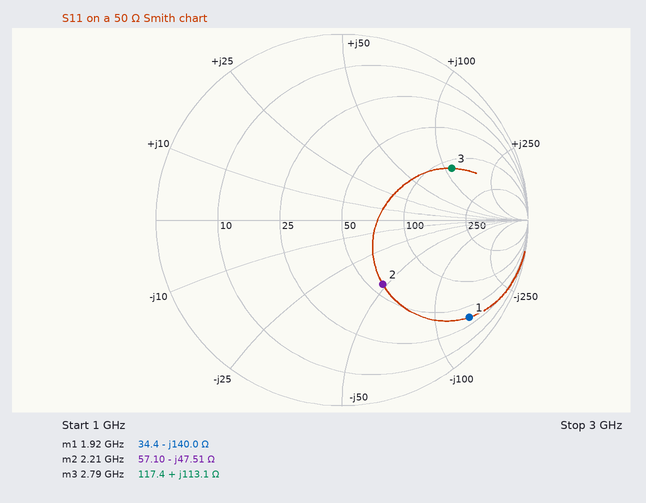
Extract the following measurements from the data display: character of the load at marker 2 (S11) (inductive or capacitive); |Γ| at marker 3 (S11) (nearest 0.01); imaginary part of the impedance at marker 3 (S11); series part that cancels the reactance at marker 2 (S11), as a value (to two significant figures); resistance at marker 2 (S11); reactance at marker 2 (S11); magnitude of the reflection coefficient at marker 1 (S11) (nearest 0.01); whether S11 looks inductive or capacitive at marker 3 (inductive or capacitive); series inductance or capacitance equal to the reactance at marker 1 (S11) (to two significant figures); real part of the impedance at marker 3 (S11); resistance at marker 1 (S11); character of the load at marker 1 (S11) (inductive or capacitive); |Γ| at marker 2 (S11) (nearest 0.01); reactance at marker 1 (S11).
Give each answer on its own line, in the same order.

capacitive
0.65
+113.1 Ω
3.4 nH
57.10 Ω
-47.51 Ω
0.86
inductive
590 fF
117.4 Ω
34.4 Ω
capacitive
0.41
-140.0 Ω
